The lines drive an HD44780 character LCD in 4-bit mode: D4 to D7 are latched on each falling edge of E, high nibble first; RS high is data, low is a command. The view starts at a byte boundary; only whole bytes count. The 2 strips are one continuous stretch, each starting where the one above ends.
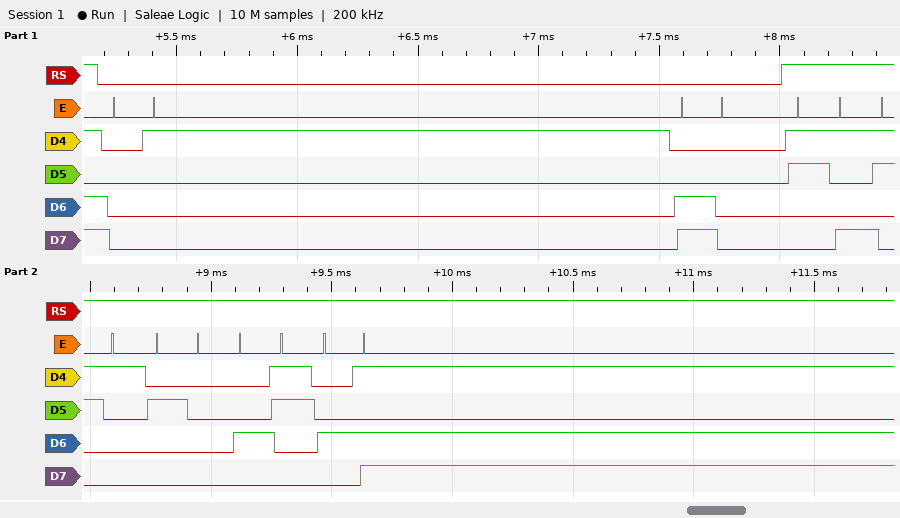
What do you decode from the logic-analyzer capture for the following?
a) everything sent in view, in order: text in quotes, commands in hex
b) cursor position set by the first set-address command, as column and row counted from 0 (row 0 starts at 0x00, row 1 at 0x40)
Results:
0x01 0xC0 "91 CM"
column 0, row 1
